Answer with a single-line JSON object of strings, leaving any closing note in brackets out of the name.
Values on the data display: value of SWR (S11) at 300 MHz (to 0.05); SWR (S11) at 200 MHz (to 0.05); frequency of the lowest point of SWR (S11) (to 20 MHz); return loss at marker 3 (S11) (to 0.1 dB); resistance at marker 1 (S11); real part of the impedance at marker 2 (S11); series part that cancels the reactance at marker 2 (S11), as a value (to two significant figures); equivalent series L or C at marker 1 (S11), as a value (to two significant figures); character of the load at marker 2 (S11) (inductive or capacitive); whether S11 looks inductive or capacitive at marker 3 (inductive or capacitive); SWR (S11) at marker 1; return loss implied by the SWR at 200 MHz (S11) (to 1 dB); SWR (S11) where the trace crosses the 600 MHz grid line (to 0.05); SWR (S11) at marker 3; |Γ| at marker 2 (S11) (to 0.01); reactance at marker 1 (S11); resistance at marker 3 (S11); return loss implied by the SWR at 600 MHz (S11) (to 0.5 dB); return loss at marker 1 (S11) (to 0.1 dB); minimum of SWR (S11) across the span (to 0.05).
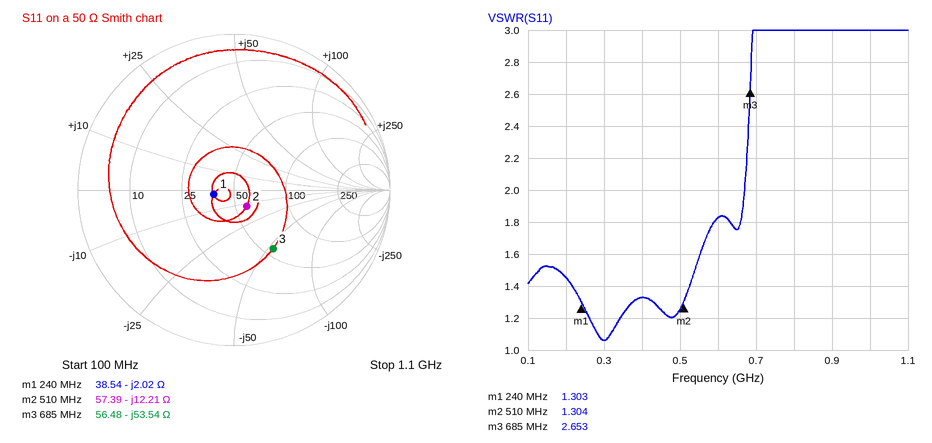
{"value of SWR (S11) at 300 MHz": "1.05", "SWR (S11) at 200 MHz": "1.45", "frequency of the lowest point of SWR (S11)": "300 MHz", "return loss at marker 3 (S11)": "6.9 dB", "resistance at marker 1": "38.54 Ω", "real part of the impedance at marker 2": "57.39 Ω", "series part that cancels the reactance at marker 2 (S11), as a value": "3.8 nH", "equivalent series L or C at marker 1 (S11), as a value": "330 pF", "character of the load at marker 2 (S11)": "capacitive", "whether S11 looks inductive or capacitive at marker 3": "capacitive", "SWR (S11) at marker 1": "1.303", "return loss implied by the SWR at 200 MHz (S11)": "15 dB", "SWR (S11) where the trace crosses the 600 MHz grid line": "1.85", "SWR (S11) at marker 3": "2.653", "|Γ| at marker 2 (S11)": "0.13", "reactance at marker 1": "-2.02 Ω", "resistance at marker 3": "56.48 Ω", "return loss implied by the SWR at 600 MHz (S11)": "10.5 dB", "return loss at marker 1 (S11)": "17.6 dB", "minimum of SWR (S11) across the span": "1.05"}
